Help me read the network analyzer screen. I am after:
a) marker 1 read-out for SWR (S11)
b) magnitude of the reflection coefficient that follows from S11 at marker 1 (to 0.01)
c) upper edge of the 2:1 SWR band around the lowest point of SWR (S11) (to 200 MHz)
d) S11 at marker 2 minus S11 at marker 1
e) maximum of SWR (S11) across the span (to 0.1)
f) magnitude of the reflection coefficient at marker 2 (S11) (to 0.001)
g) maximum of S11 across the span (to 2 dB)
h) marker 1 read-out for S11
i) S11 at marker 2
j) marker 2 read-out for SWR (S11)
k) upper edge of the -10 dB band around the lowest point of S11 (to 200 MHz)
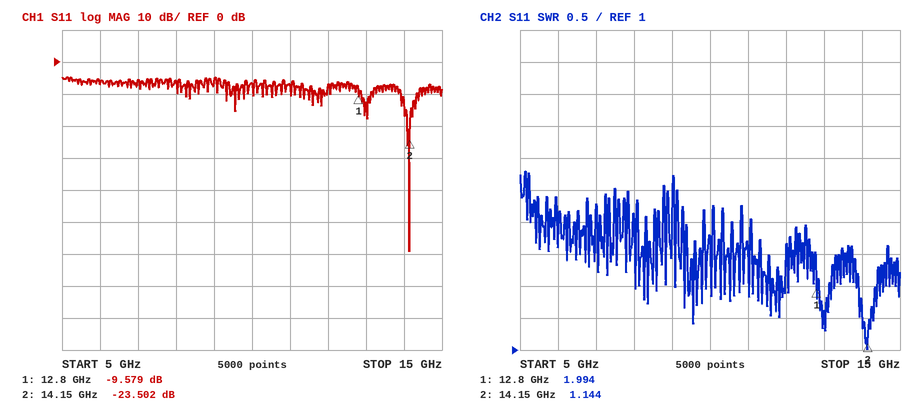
1.994
0.33
14.4 GHz
-13.923 dB
3.8
0.067
-4 dB
-9.579 dB
-23.502 dB
1.144
14.4 GHz
